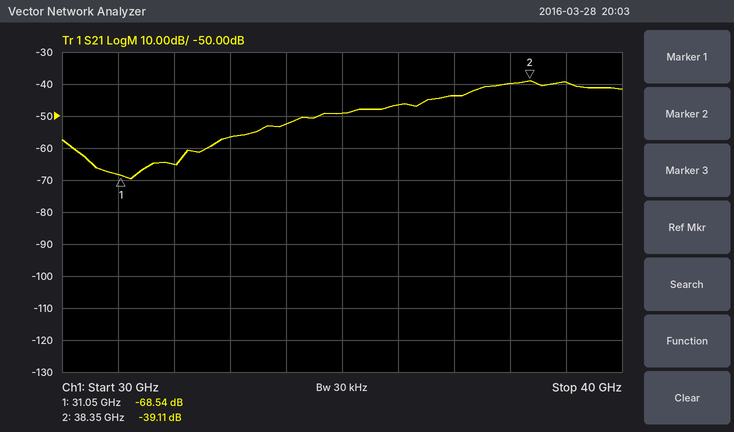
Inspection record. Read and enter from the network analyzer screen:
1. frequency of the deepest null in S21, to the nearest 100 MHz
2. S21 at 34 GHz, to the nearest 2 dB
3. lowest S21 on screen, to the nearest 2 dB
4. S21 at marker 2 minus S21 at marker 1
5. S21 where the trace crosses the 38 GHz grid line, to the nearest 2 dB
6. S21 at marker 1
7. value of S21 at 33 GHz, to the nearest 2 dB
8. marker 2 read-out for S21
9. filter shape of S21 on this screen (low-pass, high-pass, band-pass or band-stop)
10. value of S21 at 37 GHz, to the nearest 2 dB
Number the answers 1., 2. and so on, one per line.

1. 31.2 GHz
2. -52 dB
3. -70 dB
4. 29.43 dB
5. -40 dB
6. -68.54 dB
7. -56 dB
8. -39.11 dB
9. high-pass
10. -44 dB
